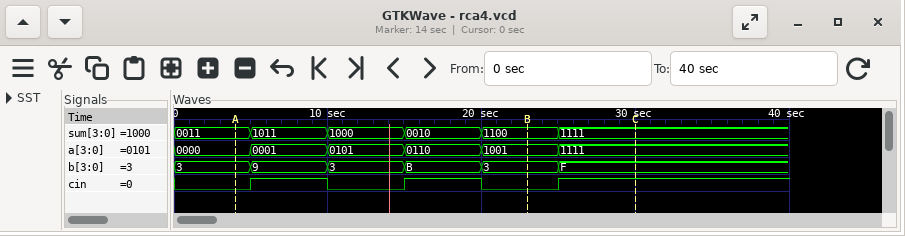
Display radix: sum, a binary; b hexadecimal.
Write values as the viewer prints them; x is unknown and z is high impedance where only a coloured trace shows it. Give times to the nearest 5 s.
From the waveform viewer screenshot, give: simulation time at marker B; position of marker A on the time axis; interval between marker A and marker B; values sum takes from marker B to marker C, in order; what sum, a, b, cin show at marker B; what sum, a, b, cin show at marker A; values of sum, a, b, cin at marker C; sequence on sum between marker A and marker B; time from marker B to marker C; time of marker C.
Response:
25 s
5 s
20 s
1100, 1111
sum=1100, a=1001, b=3, cin=0
sum=0011, a=0000, b=3, cin=0
sum=1111, a=1111, b=F, cin=1
0011, 1011, 1000, 0010, 1100
5 s
30 s
